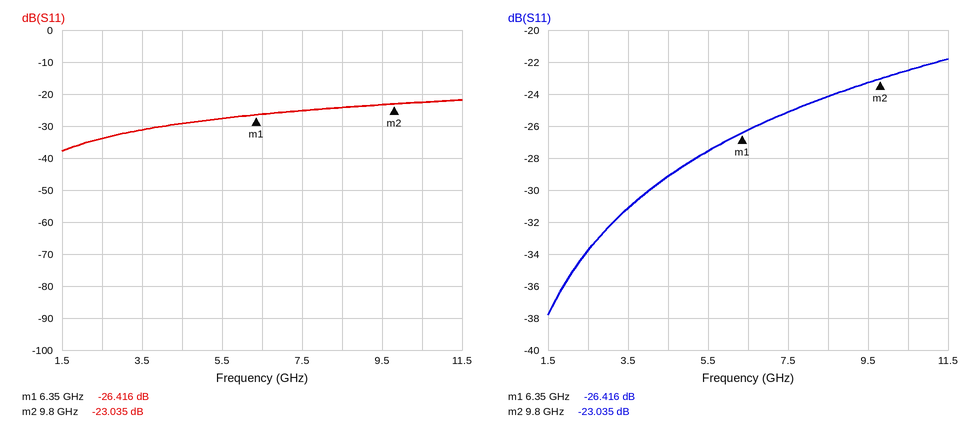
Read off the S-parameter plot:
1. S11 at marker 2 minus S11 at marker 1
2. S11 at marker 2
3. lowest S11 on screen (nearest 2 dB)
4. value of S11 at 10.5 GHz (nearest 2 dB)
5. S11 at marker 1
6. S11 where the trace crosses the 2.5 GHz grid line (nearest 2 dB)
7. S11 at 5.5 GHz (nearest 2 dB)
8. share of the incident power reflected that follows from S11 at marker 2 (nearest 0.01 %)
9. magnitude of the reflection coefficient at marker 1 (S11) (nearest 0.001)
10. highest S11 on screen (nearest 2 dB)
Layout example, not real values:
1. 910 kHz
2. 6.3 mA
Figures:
1. 3.381 dB
2. -23.035 dB
3. -38 dB
4. -22 dB
5. -26.416 dB
6. -34 dB
7. -28 dB
8. 0.50 %
9. 0.048
10. -22 dB
